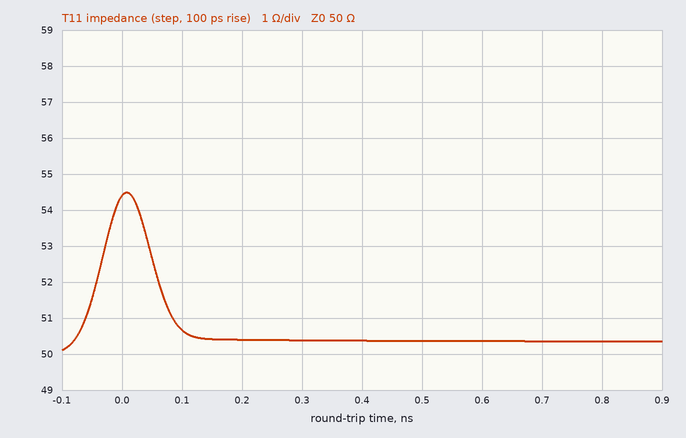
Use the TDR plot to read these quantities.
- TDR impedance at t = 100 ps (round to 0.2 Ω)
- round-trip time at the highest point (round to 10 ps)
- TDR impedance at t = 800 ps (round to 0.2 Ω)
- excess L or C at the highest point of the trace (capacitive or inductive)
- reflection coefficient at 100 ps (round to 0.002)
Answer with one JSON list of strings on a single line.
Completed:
["50.6 Ω", "10 ps", "50.4 Ω", "inductive", "+0.006"]
